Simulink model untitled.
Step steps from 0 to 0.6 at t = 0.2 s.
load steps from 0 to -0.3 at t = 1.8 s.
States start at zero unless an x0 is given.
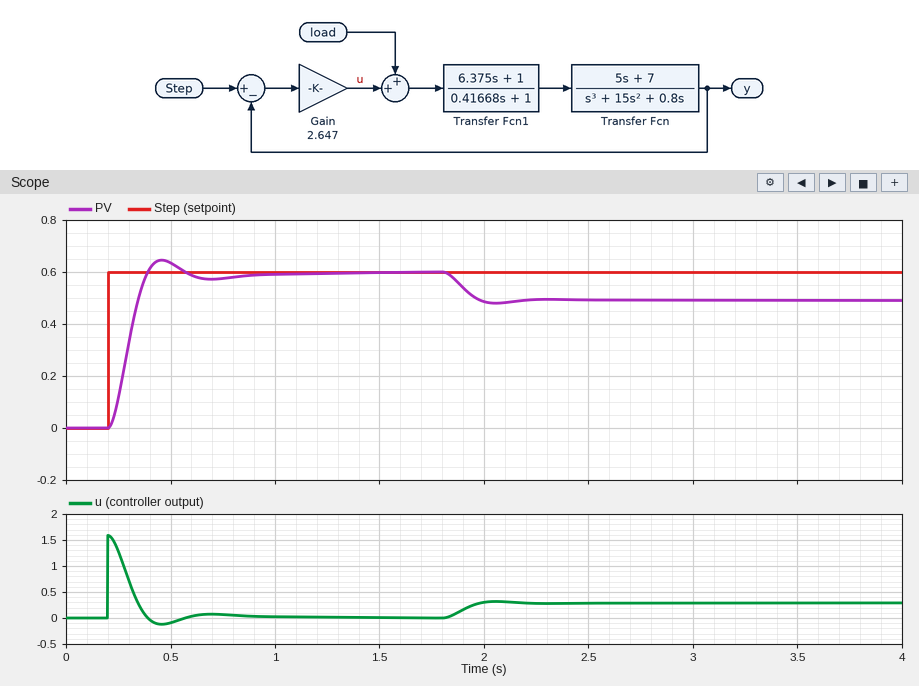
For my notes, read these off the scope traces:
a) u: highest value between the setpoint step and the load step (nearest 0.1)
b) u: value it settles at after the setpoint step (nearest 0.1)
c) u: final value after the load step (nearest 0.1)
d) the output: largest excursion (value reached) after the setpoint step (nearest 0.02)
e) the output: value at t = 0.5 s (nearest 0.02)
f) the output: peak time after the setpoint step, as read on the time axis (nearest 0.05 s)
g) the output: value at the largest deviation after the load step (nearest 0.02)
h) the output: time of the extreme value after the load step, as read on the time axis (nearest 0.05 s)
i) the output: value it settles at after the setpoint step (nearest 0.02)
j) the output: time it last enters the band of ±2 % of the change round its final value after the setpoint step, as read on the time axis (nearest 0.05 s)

1.6
0.0
0.3
0.64
0.64
0.45 s
0.48
2.05 s
0.60
0.90 s
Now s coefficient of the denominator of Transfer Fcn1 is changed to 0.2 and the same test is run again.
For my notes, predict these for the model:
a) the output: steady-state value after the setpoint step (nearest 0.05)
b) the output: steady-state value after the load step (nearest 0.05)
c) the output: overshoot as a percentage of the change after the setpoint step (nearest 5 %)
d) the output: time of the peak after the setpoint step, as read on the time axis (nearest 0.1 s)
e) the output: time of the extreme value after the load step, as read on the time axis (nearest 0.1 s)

0.60
0.50
10 %
0.4 s
2.0 s
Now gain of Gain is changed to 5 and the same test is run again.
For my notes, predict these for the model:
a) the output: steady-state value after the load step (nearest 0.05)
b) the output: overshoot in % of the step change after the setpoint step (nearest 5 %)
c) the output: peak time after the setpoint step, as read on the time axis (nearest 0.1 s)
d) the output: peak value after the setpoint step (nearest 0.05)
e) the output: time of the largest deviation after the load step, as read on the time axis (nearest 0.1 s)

0.55
20 %
0.4 s
0.75
2.0 s
